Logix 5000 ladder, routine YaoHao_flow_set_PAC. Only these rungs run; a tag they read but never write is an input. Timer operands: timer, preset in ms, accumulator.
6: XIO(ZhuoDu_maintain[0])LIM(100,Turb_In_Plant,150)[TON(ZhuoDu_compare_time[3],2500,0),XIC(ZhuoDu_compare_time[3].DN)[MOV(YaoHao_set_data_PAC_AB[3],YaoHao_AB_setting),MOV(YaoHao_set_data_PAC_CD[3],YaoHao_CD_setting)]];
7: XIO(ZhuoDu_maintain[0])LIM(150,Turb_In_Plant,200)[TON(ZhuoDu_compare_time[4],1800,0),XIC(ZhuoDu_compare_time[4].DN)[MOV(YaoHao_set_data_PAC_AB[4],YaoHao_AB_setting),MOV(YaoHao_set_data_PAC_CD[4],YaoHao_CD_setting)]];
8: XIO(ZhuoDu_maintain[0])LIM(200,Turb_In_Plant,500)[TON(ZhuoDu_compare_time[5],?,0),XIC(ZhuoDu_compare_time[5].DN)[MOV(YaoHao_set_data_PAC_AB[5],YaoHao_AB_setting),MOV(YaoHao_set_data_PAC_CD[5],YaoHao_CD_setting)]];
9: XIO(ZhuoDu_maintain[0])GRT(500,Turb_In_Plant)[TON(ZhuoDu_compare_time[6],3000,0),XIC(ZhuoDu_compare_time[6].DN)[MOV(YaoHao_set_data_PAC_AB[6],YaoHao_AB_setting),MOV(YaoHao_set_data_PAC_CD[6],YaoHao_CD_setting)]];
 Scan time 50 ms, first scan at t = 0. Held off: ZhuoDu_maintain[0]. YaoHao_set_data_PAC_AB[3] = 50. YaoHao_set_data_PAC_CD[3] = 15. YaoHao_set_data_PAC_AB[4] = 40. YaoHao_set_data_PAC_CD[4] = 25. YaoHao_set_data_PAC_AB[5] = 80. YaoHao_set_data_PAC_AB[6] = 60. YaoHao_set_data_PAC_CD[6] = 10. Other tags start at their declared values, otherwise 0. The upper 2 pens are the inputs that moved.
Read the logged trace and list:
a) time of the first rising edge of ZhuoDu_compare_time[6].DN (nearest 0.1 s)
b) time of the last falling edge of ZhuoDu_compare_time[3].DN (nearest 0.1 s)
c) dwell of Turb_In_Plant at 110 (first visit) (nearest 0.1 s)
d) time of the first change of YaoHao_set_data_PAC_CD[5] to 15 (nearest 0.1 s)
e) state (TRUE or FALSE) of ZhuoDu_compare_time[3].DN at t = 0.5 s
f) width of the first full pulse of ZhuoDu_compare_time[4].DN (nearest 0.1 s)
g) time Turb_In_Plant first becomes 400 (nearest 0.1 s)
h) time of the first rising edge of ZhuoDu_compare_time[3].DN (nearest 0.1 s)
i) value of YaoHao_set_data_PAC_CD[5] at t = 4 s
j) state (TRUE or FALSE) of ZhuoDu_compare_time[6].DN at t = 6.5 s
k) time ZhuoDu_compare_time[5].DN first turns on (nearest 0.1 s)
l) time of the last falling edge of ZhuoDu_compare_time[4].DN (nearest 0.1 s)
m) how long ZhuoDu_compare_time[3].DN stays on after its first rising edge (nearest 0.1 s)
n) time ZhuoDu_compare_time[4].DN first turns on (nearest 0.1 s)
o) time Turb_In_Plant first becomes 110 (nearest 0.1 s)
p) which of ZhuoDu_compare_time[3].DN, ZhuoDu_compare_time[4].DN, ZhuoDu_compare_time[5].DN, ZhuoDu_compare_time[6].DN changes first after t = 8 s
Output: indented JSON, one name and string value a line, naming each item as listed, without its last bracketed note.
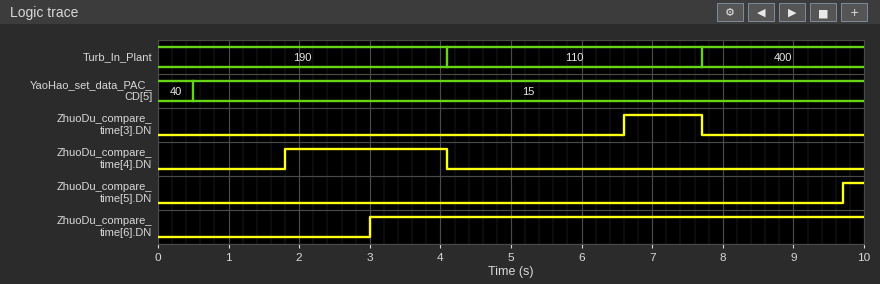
{
  "time of the first rising edge of ZhuoDu_compare_time[6].DN": "3.0 s",
  "time of the last falling edge of ZhuoDu_compare_time[3].DN": "7.7 s",
  "dwell of Turb_In_Plant at 110 (first visit)": "3.6 s",
  "time of the first change of YaoHao_set_data_PAC_CD[5] to 15": "0.5 s",
  "state (TRUE or FALSE) of ZhuoDu_compare_time[3].DN at t = 0.5 s": "FALSE",
  "width of the first full pulse of ZhuoDu_compare_time[4].DN": "2.3 s",
  "time Turb_In_Plant first becomes 400": "7.7 s",
  "time of the first rising edge of ZhuoDu_compare_time[3].DN": "6.6 s",
  "value of YaoHao_set_data_PAC_CD[5] at t = 4 s": "15",
  "state (TRUE or FALSE) of ZhuoDu_compare_time[6].DN at t = 6.5 s": "TRUE",
  "time ZhuoDu_compare_time[5].DN first turns on": "9.7 s",
  "time of the last falling edge of ZhuoDu_compare_time[4].DN": "4.1 s",
  "how long ZhuoDu_compare_time[3].DN stays on after its first rising edge": "1.1 s",
  "time ZhuoDu_compare_time[4].DN first turns on": "1.8 s",
  "time Turb_In_Plant first becomes 110": "4.1 s",
  "which of ZhuoDu_compare_time[3].DN, ZhuoDu_compare_time[4].DN, ZhuoDu_compare_time[5].DN, ZhuoDu_compare_time[6].DN changes first after t = 8 s": "ZhuoDu_compare_time[5].DN"
}
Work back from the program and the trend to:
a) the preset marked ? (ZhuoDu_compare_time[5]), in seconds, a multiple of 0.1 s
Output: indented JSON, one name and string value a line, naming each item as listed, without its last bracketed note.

{
  "the preset marked ? (ZhuoDu_compare_time[5]), in seconds, a multiple of 0.1 s": "2.0 s"
}
